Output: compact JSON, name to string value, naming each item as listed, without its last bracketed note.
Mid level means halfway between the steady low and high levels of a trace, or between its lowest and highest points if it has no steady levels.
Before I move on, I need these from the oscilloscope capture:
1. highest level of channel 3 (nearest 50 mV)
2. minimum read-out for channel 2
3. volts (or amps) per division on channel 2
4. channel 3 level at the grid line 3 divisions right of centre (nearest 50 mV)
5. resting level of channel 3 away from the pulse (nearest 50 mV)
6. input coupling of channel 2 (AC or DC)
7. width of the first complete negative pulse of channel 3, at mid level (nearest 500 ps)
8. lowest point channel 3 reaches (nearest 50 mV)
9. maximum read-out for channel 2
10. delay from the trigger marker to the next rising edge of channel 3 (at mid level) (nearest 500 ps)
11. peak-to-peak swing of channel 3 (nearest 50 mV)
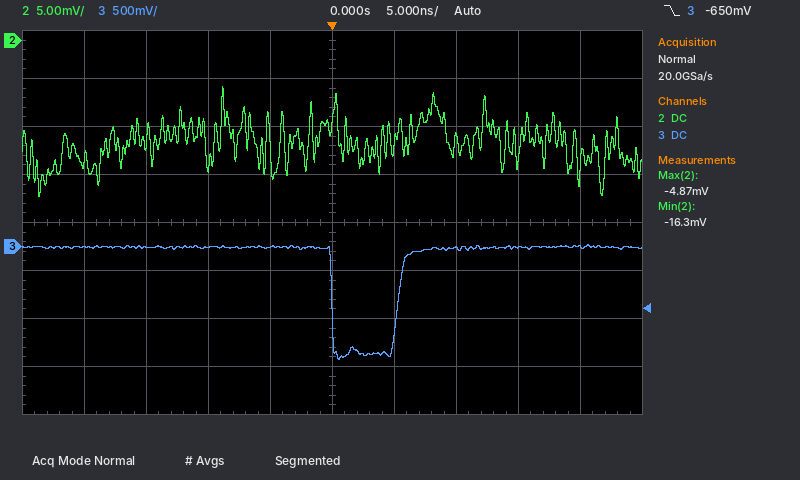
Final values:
{"highest level of channel 3": "0 mV", "minimum read-out for channel 2": "-16.3 mV", "volts (or amps) per division on channel 2": "5 mV", "channel 3 level at the grid line 3 divisions right of centre": "0 mV", "resting level of channel 3 away from the pulse": "0 mV", "input coupling of channel 2": "DC", "width of the first complete negative pulse of channel 3, at mid level": "5.5 ns", "lowest point channel 3 reaches": "-1.20 V", "maximum read-out for channel 2": "-4.87 mV", "delay from the trigger marker to the next rising edge of channel 3 (at mid level)": "5.5 ns", "peak-to-peak swing of channel 3": "1.20 V"}
